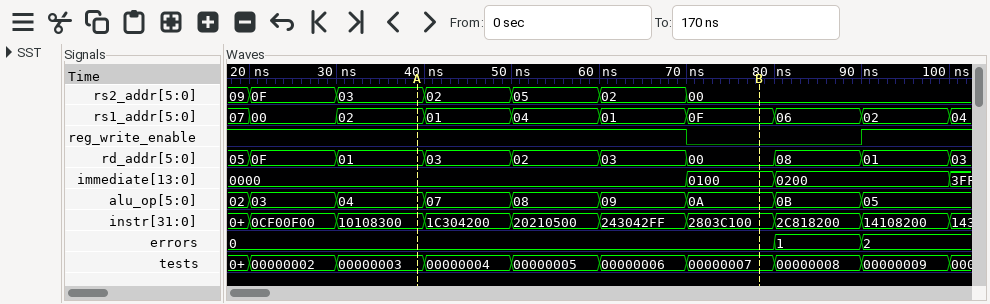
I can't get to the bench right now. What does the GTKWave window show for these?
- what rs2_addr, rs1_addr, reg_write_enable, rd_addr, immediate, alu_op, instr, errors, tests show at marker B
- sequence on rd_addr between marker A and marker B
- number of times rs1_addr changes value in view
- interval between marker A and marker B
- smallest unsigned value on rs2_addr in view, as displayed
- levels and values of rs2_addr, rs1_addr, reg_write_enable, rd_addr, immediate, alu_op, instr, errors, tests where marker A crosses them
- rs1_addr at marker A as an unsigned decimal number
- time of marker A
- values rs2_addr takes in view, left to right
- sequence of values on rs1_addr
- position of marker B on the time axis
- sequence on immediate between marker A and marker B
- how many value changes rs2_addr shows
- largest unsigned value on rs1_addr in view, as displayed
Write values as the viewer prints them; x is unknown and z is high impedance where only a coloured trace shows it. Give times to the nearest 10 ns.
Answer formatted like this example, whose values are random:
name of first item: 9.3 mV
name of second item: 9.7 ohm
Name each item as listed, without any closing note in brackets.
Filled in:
what rs2_addr, rs1_addr, reg_write_enable, rd_addr, immediate, alu_op, instr, errors, tests show at marker B: rs2_addr=00, rs1_addr=0F, reg_write_enable=0, rd_addr=00, immediate=0100, alu_op=0A, instr=2803C100, errors=0, tests=00000007
sequence on rd_addr between marker A and marker B: 01, 03, 02, 03, 00
number of times rs1_addr changes value in view: 9
interval between marker A and marker B: 40 ns
smallest unsigned value on rs2_addr in view, as displayed: 00
levels and values of rs2_addr, rs1_addr, reg_write_enable, rd_addr, immediate, alu_op, instr, errors, tests where marker A crosses them: rs2_addr=03, rs1_addr=02, reg_write_enable=1, rd_addr=01, immediate=0000, alu_op=04, instr=10108300, errors=0, tests=00000003
rs1_addr at marker A as an unsigned decimal number: 2
time of marker A: 40 ns
values rs2_addr takes in view, left to right: 09, 0F, 03, 02, 05, 02, 00
sequence of values on rs1_addr: 07, 00, 02, 01, 04, 01, 0F, 06, 02, 04
position of marker B on the time axis: 80 ns
sequence on immediate between marker A and marker B: 0000, 0100
how many value changes rs2_addr shows: 6
largest unsigned value on rs1_addr in view, as displayed: 0F
